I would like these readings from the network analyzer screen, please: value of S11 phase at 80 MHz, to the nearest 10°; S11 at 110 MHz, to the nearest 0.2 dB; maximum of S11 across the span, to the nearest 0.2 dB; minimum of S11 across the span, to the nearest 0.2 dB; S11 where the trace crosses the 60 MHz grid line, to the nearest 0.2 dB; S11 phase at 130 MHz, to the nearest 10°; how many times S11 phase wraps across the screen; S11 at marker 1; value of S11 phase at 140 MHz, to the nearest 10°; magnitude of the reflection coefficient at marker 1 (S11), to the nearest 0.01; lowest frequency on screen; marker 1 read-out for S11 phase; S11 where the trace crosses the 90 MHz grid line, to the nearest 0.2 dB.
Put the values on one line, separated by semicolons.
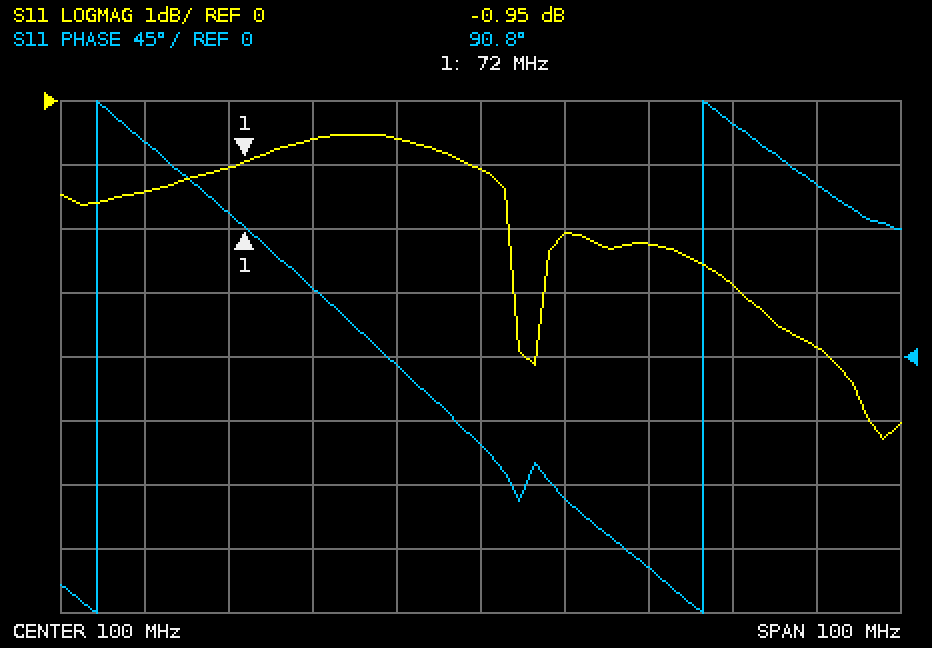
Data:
50°; -2.0 dB; -0.6 dB; -5.2 dB; -1.4 dB; 160°; 2; -0.95 dB; 120°; 0.90; 50 MHz; 90.8°; -0.6 dB
